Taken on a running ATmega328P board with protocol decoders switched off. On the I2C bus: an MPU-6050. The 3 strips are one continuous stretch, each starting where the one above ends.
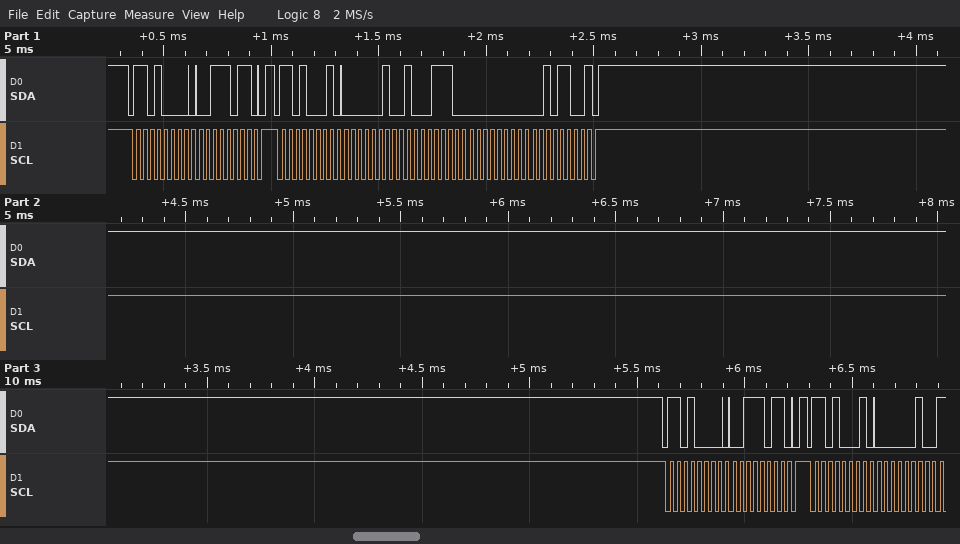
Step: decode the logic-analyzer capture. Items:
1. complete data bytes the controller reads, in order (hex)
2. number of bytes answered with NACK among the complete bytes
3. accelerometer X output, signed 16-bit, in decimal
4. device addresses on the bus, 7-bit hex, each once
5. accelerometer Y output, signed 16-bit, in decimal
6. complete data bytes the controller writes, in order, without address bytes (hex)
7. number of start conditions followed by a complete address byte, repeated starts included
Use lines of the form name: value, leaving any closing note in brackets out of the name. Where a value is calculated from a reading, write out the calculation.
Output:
complete data bytes the controller reads, in order: 02 8E 00 2C 02
number of bytes answered with NACK among the complete bytes: 1
accelerometer X output, signed 16-bit, in decimal: 0x028E = 654
device addresses on the bus, 7-bit hex, each once: 0x68
accelerometer Y output, signed 16-bit, in decimal: 0x002C = 44
complete data bytes the controller writes, in order, without address bytes: 3B 3B
number of start conditions followed by a complete address byte, repeated starts included: 4
